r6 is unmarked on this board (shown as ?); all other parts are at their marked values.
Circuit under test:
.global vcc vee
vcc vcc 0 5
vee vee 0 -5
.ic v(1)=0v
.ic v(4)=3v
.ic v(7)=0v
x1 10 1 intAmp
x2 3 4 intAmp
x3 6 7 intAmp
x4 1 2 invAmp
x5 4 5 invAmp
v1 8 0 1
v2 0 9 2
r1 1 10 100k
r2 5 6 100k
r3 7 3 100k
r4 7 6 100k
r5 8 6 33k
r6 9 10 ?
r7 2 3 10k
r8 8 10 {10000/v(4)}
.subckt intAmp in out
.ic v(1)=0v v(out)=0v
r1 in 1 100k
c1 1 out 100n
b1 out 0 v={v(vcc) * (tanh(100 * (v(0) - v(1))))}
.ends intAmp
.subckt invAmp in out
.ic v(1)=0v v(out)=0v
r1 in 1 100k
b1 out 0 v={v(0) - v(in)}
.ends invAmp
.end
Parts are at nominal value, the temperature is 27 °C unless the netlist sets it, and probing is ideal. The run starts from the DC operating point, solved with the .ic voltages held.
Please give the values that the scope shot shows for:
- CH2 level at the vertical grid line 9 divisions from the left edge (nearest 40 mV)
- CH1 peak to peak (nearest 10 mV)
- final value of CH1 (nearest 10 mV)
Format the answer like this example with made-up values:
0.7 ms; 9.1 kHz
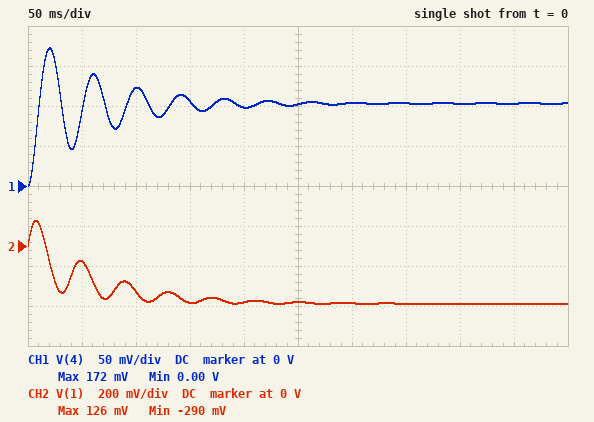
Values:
-280 mV; 170 mV; 100 mV
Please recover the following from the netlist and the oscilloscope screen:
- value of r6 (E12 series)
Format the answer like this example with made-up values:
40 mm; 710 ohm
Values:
270 kΩ
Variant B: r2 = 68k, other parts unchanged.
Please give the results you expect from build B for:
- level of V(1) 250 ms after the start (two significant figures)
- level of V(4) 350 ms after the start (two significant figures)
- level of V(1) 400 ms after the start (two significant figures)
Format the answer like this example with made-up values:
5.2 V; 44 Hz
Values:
-270 mV; 100 mV; -280 mV
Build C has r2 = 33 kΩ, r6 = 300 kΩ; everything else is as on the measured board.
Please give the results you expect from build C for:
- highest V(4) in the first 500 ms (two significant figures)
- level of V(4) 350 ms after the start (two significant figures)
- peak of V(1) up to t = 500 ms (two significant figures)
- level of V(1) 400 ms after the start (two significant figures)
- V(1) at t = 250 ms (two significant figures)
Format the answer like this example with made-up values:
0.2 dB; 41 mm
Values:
150 mV; 93 mV; 120 mV; -270 mV; -260 mV
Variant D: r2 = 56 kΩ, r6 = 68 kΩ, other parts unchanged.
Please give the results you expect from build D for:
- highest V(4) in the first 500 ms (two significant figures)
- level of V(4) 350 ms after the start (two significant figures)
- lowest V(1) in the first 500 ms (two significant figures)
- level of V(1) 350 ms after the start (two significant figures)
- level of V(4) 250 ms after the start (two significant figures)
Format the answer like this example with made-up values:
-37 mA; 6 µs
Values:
680 mV; 310 mV; -480 mV; -210 mV; 370 mV
